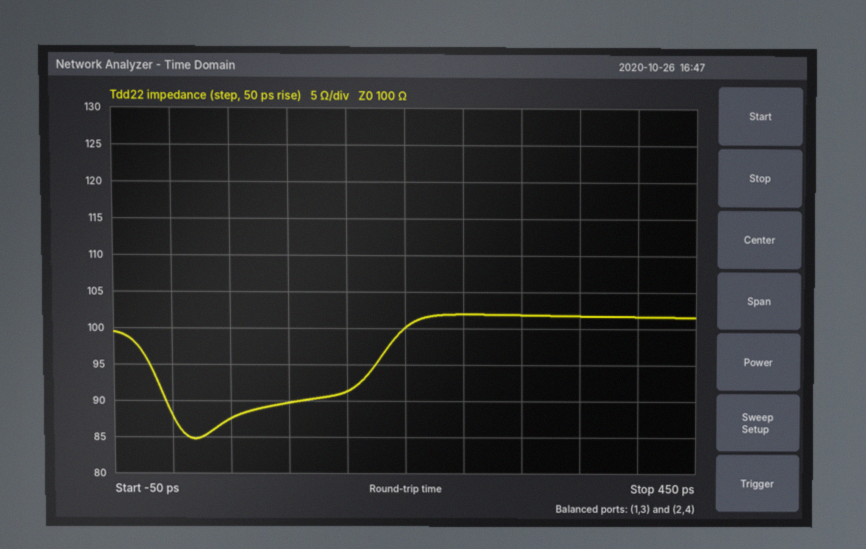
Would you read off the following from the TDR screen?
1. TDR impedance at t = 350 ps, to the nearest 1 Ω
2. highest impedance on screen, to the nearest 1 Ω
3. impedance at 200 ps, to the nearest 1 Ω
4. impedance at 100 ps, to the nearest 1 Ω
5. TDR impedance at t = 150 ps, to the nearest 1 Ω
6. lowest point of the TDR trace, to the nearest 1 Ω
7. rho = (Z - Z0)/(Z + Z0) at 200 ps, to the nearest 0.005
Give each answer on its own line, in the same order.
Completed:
102 Ω
102 Ω
100 Ω
90 Ω
91 Ω
85 Ω
0.000
